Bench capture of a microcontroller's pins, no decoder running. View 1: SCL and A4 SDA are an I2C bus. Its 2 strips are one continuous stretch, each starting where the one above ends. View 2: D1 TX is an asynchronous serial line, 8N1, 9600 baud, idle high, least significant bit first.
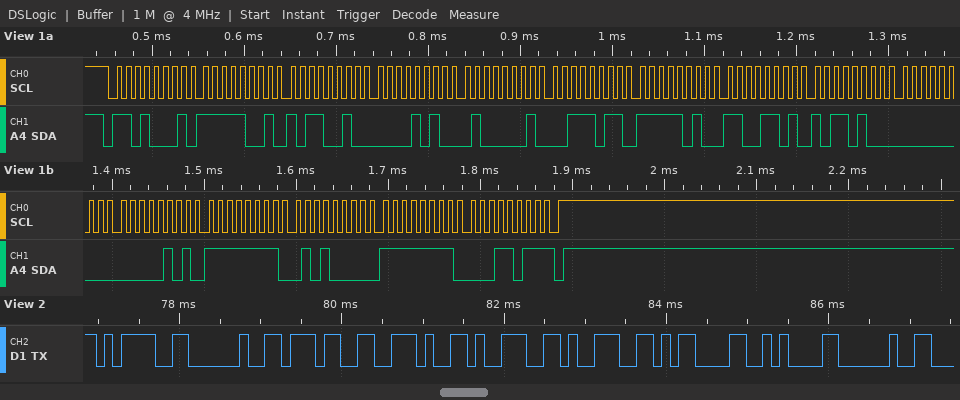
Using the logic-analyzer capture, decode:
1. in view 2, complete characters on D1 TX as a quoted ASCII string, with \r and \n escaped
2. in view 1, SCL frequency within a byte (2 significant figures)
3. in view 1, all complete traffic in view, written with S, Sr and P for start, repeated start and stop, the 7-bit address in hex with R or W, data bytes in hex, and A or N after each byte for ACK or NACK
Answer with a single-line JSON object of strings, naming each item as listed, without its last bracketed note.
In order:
{"in view 2, complete characters on D1 TX as a quoted ASCII string, with \\r and \\n escaped": "\"= 7.99\\r\\n \"", "in view 1, SCL frequency within a byte": "100 kHz", "in view 1, all complete traffic in view, written with S, Sr and P for start, repeated start and stop, the 7-bit address in hex with R or W, data bytes in hex, and A or N after each byte for ACK or NACK": "S 68R A F9 A B2 A 0A A 41 A 3B A FA A CD A B4 A 00 A 05 A FF A 50 A FF A 1B N P"}
